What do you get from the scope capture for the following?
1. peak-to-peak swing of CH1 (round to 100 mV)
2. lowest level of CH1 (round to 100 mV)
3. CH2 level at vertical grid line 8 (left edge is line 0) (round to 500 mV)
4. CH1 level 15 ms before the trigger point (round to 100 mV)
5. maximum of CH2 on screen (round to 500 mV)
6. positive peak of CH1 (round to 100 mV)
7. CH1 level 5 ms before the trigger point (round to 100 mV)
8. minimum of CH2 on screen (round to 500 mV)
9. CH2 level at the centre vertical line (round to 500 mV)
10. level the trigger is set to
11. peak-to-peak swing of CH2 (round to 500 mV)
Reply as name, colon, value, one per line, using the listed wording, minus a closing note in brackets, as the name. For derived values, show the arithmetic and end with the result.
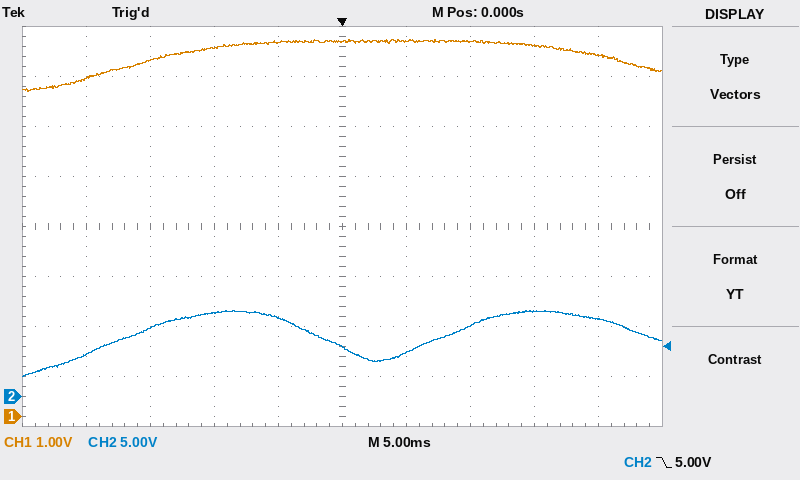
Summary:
peak-to-peak swing of CH1: 7.5 V − (6.5 V) = 1.0 V
lowest level of CH1: 6.5 V
CH2 level at vertical grid line 8 (left edge is line 0): 8.5 V
CH1 level 15 ms before the trigger point: 7.1 V
maximum of CH2 on screen: 8.5 V
positive peak of CH1: 7.5 V
CH1 level 5 ms before the trigger point: 7.5 V
minimum of CH2 on screen: 2.0 V
CH2 level at the centre vertical line: 5.0 V
level the trigger is set to: 5.00 V
peak-to-peak swing of CH2: 8.5 V − (2.0 V) = 6.5 V
